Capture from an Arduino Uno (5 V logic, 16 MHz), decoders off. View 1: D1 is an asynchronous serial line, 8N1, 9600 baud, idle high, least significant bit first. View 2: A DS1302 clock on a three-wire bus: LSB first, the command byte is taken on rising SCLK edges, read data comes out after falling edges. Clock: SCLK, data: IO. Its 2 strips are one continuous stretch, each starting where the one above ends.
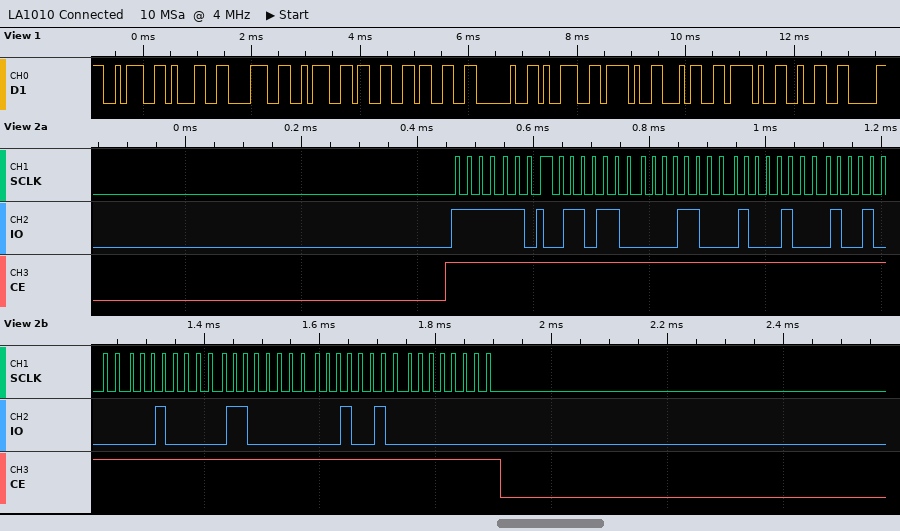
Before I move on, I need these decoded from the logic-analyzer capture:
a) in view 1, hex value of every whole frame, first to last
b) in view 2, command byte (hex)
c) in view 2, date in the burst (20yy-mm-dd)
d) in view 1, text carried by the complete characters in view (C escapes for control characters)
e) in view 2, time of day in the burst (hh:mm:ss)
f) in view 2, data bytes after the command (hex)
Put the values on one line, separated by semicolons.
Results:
3A 31 38 3A 33 33 20 39 2F 34 2F 32; 0xBF; 2024-04-09; ":18:33 9/4/2"; 11:18:36; 36 18 11 09 04 03 24 00
